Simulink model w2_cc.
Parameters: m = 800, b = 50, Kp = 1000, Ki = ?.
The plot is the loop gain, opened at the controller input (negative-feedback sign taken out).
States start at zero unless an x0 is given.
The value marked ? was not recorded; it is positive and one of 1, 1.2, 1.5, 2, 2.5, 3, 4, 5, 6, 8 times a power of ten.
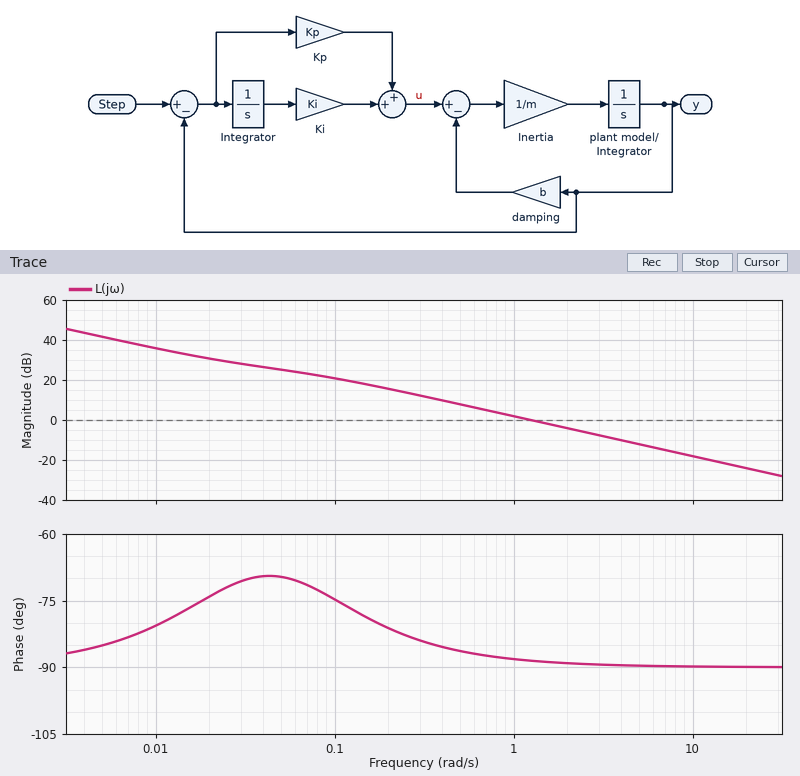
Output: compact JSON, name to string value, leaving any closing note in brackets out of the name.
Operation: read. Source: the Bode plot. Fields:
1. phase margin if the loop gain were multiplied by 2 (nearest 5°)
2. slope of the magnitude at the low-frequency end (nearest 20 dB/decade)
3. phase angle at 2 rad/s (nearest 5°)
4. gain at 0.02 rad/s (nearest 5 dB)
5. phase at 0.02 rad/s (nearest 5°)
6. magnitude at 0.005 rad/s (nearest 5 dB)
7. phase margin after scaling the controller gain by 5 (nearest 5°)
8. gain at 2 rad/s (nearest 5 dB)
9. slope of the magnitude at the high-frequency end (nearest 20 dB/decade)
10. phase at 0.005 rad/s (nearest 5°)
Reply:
{"phase margin if the loop gain were multiplied by 2": "90°", "slope of the magnitude at the low-frequency end": "-20 dB/decade", "phase angle at 2 rad/s": "-90°", "gain at 0.02 rad/s": "30 dB", "phase at 0.02 rad/s": "-75°", "magnitude at 0.005 rad/s": "40 dB", "phase margin after scaling the controller gain by 5": "90°", "gain at 2 rad/s": "-5 dB", "slope of the magnitude at the high-frequency end": "-20 dB/decade", "phase at 0.005 rad/s": "-85°"}
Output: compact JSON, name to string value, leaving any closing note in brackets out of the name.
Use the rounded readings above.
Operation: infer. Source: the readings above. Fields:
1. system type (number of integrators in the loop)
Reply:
{"system type": "1"}
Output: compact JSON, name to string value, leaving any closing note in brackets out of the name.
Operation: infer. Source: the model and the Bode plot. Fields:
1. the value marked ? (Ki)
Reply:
{"the value marked ?": "30"}
